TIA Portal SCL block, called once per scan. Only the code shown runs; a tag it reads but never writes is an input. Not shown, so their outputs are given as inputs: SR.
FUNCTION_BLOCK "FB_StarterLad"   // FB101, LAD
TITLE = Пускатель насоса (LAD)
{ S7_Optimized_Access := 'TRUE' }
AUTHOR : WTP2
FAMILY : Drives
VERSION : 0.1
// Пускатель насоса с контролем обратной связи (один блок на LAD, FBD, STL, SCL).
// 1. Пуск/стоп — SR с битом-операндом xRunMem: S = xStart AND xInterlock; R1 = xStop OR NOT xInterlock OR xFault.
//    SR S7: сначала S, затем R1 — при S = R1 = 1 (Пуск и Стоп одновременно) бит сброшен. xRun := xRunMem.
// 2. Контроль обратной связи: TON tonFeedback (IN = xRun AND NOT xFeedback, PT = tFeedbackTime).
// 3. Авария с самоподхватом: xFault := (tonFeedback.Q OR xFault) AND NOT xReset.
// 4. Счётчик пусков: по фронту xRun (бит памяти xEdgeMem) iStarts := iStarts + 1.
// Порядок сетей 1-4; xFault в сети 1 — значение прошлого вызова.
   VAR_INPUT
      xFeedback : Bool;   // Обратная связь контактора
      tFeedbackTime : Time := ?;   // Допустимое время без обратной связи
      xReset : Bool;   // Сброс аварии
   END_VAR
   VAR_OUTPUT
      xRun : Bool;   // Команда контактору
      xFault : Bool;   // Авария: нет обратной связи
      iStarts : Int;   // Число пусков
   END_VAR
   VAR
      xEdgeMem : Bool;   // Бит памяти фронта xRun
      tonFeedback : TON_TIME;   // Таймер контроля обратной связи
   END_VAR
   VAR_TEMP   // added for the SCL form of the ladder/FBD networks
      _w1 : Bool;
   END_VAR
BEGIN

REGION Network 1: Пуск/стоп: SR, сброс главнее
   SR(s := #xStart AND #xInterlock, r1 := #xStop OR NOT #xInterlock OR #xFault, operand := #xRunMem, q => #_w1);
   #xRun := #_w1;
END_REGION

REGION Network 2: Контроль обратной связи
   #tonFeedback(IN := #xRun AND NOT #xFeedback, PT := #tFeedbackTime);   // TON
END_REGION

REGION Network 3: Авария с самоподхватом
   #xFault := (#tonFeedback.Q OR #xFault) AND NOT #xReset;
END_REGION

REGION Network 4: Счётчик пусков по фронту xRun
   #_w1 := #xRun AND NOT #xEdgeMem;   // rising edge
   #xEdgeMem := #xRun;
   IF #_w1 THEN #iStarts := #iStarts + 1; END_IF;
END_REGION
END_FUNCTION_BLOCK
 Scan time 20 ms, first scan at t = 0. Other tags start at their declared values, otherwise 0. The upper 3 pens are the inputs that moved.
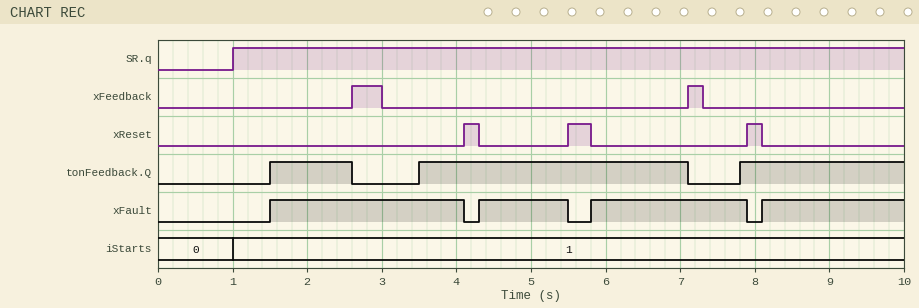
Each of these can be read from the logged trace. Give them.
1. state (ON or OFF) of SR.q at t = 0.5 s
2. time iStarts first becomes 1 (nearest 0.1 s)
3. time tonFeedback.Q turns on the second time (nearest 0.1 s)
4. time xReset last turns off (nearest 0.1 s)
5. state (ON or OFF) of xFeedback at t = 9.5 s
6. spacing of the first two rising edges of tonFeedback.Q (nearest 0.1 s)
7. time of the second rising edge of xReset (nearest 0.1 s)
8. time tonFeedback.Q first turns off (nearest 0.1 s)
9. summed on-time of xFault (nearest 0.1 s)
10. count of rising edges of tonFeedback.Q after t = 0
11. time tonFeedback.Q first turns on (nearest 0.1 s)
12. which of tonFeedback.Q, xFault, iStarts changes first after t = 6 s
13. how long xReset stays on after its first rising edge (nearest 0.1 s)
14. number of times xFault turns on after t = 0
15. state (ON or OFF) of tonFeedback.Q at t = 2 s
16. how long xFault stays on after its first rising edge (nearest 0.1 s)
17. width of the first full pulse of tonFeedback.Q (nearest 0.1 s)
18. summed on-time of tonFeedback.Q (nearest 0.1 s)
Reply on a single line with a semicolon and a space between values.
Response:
OFF; 1.0 s; 3.5 s; 8.1 s; OFF; 2.0 s; 5.5 s; 2.6 s; 7.8 s; 3; 1.5 s; tonFeedback.Q; 0.2 s; 4; ON; 2.6 s; 1.1 s; 6.9 s
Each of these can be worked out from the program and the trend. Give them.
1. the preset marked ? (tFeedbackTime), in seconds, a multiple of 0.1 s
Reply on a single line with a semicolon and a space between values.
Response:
0.5 s
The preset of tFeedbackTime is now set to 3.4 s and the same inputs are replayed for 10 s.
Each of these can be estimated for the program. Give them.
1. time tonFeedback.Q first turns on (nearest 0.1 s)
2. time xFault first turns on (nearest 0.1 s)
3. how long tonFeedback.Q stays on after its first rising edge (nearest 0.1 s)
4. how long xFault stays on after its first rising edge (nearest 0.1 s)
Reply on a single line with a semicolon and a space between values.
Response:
6.4 s; 6.4 s; 0.7 s; 1.5 s
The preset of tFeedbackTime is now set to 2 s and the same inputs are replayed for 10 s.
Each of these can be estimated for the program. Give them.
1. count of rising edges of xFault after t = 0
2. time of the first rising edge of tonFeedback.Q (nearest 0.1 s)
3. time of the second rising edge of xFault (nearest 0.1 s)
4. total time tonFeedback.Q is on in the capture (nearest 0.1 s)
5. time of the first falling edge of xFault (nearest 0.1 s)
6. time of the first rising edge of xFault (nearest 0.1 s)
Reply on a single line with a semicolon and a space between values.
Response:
3; 5.0 s; 5.8 s; 2.8 s; 5.5 s; 5.0 s
